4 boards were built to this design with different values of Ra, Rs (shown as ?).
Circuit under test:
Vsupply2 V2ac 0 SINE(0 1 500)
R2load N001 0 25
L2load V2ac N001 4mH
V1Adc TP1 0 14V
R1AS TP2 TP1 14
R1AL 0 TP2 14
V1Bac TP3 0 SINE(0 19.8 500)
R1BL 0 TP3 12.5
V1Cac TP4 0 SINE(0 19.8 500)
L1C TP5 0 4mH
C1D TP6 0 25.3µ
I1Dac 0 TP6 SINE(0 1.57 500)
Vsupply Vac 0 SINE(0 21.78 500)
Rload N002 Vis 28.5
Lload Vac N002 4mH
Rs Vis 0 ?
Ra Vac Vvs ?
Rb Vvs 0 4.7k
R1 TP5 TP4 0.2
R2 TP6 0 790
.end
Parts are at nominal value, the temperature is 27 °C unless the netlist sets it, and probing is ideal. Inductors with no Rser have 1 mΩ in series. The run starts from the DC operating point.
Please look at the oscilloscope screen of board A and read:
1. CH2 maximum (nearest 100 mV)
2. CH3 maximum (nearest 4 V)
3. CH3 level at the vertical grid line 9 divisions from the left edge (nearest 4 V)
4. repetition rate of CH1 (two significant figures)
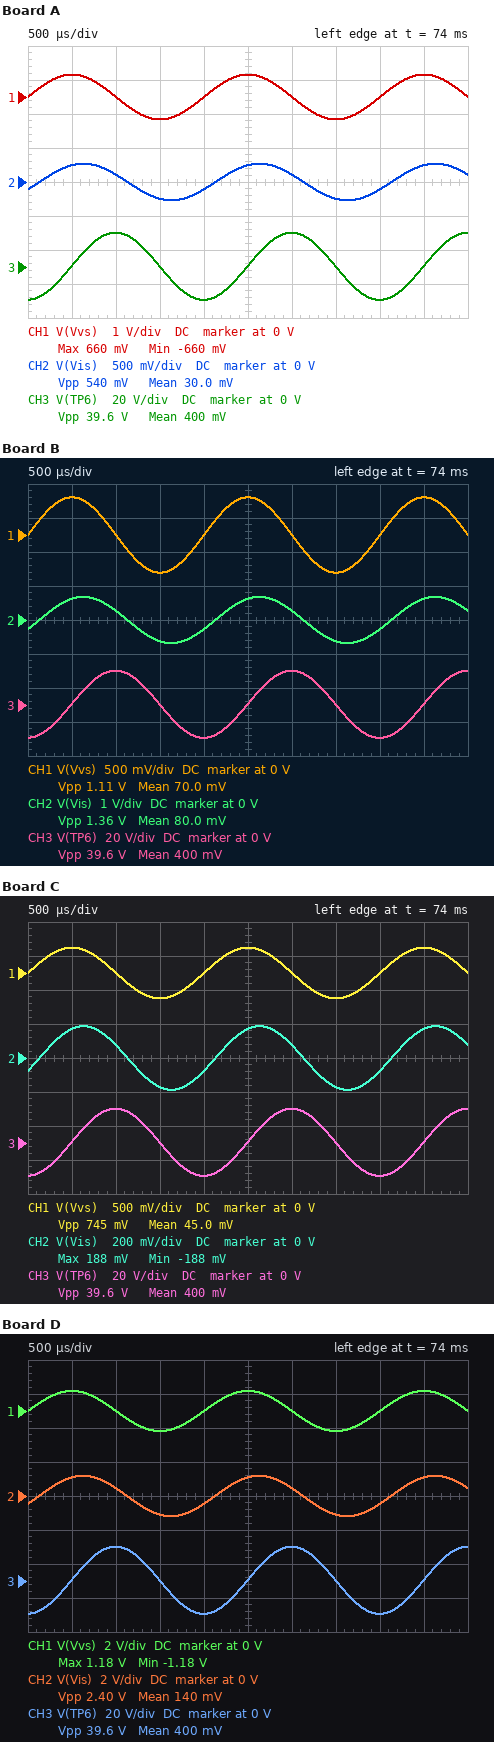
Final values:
300 mV
20 V
0 V
500 Hz
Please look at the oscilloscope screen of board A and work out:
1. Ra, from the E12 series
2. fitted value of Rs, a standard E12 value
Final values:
150 kΩ
0.39 Ω
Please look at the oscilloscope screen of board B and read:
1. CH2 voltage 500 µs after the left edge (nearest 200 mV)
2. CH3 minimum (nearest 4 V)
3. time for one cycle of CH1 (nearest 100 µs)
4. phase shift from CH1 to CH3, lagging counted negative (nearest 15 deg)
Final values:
600 mV
-20 V
2.0 ms
-90 deg
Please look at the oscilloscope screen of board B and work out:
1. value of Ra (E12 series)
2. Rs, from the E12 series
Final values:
180 kΩ
1 Ω
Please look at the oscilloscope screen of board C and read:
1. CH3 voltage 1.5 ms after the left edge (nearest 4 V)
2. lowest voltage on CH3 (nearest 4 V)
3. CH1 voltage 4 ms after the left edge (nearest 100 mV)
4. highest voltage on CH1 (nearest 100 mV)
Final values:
0 V
-20 V
0 V
400 mV
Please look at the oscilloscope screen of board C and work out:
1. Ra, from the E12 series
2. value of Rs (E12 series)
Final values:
270 kΩ
0.27 Ω
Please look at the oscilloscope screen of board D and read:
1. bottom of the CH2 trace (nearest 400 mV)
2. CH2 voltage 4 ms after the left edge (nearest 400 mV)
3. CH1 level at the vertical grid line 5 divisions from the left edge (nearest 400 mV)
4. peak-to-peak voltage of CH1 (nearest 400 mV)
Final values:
-1.2 V
-400 mV
1.2 V
2.4 V
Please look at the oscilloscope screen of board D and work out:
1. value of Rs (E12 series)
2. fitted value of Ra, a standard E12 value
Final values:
1.8 Ω
82 kΩ
